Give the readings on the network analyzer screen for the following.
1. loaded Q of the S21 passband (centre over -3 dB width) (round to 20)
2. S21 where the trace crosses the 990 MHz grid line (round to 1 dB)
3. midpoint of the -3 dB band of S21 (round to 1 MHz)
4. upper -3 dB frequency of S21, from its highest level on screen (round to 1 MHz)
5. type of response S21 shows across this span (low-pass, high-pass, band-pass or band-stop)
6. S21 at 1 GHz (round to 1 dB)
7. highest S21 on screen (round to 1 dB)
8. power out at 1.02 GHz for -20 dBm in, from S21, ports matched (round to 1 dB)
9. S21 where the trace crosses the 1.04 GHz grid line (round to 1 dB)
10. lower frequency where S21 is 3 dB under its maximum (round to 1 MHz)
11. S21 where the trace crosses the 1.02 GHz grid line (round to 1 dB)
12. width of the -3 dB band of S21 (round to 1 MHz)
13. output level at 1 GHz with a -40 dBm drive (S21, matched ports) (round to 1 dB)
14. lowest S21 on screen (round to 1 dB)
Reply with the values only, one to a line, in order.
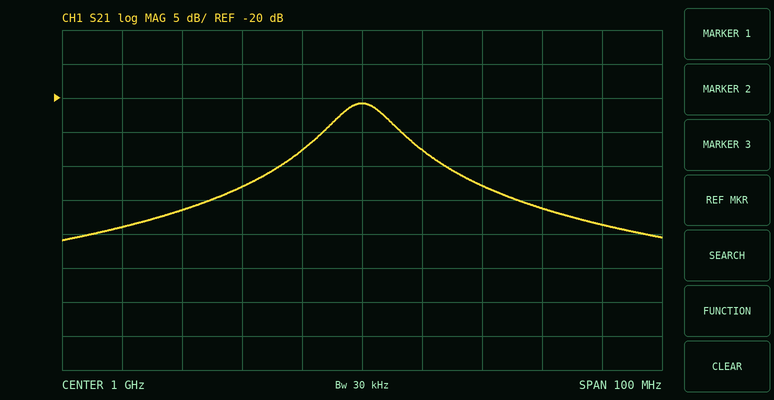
100
-28 dB
1.000 GHz
1.005 GHz
band-pass
-21 dB
-21 dB
-53 dBm
-39 dB
995 MHz
-33 dB
10 MHz
-61 dBm
-41 dB
